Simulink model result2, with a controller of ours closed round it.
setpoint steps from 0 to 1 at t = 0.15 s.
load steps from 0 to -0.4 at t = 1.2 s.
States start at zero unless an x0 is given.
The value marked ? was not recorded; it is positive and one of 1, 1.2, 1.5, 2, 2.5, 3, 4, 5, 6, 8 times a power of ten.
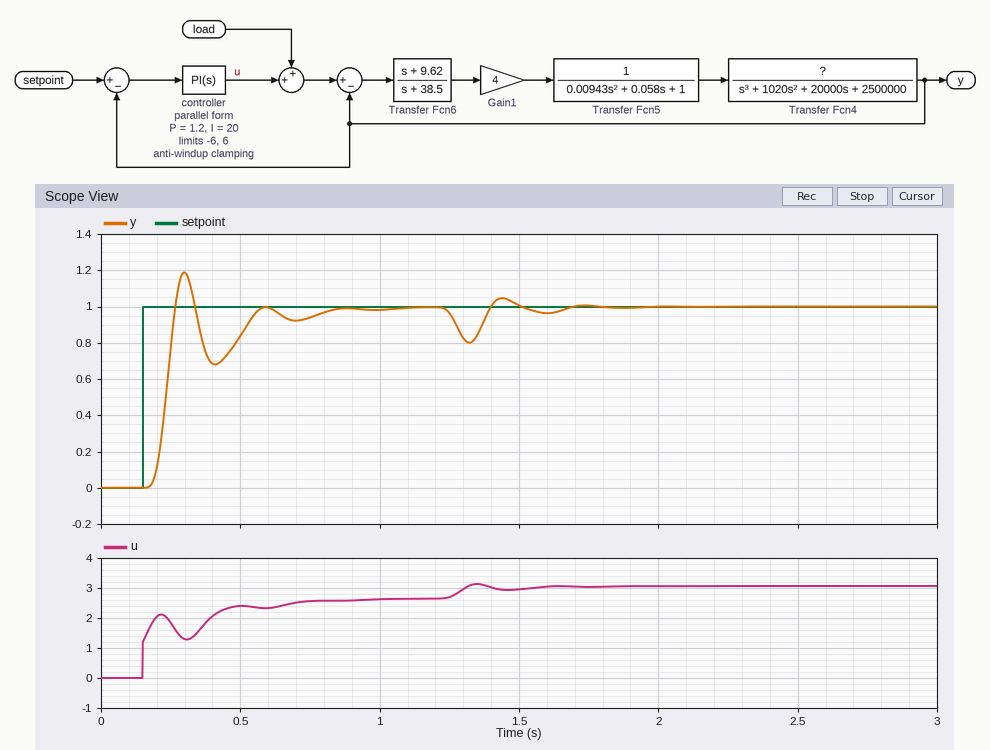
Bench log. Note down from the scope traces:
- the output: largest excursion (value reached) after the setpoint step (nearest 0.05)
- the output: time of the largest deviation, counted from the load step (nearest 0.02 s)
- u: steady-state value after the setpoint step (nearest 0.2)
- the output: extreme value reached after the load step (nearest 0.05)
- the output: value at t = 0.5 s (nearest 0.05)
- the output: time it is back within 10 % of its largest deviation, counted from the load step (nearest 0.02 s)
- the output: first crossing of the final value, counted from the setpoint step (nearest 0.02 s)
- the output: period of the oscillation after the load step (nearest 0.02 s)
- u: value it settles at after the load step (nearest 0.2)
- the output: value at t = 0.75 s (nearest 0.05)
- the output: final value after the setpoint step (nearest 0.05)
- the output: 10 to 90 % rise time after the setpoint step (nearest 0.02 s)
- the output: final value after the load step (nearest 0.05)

1.20
0.12 s
2.6
0.80
0.85
0.46 s
0.12 s
0.28 s
3.0
0.95
1.00
0.06 s
1.00
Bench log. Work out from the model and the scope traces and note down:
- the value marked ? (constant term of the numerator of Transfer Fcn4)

1.5e+06
